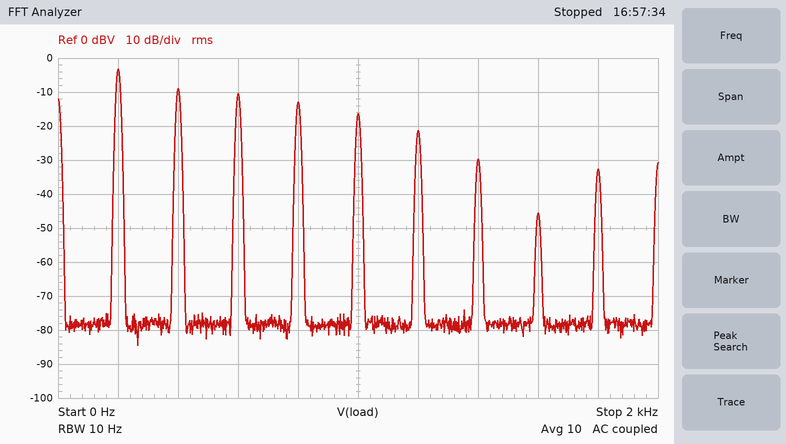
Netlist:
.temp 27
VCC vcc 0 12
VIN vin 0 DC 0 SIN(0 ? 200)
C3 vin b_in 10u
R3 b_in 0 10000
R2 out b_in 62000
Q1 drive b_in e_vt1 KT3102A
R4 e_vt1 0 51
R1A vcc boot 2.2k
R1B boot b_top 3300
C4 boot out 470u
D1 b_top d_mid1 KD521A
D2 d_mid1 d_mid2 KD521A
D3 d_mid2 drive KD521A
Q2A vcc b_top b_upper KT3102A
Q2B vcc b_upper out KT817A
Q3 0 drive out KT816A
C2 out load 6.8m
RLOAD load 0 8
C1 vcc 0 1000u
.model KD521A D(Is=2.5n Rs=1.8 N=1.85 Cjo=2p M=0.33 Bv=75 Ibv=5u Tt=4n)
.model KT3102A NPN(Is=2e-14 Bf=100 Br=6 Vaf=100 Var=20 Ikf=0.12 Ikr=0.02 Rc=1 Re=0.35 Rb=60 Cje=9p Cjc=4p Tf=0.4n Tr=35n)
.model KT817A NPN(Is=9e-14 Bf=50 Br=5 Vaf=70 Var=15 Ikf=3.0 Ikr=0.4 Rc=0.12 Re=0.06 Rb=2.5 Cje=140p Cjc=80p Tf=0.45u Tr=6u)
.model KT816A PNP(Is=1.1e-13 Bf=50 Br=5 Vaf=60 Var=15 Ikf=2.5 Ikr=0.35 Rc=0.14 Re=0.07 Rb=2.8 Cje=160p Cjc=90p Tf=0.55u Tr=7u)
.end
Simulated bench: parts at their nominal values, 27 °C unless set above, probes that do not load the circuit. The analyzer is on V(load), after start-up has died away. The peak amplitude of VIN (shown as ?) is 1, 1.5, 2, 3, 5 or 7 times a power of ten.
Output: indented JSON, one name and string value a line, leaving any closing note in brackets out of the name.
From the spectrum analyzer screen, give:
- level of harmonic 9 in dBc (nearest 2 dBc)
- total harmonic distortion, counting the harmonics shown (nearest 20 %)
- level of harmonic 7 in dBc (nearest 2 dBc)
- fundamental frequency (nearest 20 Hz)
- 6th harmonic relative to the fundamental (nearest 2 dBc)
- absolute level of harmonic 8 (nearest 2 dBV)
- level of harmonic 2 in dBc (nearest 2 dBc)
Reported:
{
  "level of harmonic 9 in dBc": "-30 dBc",
  "total harmonic distortion, counting the harmonics shown": "80 %",
  "level of harmonic 7 in dBc": "-26 dBc",
  "fundamental frequency": "200 Hz",
  "6th harmonic relative to the fundamental": "-18 dBc",
  "absolute level of harmonic 8": "-46 dBV",
  "level of harmonic 2 in dBc": "-6 dBc"
}
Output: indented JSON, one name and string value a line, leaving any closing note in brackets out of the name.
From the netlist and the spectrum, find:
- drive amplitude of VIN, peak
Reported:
{
  "drive amplitude of VIN, peak": "70 mV"
}
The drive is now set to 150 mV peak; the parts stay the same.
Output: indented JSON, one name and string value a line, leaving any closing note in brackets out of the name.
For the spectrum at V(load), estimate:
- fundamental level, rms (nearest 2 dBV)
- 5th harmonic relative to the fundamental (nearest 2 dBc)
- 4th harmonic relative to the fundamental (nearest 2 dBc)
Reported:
{
  "fundamental level, rms": "4 dBV",
  "5th harmonic relative to the fundamental": "-22 dBc",
  "4th harmonic relative to the fundamental": "-14 dBc"
}
